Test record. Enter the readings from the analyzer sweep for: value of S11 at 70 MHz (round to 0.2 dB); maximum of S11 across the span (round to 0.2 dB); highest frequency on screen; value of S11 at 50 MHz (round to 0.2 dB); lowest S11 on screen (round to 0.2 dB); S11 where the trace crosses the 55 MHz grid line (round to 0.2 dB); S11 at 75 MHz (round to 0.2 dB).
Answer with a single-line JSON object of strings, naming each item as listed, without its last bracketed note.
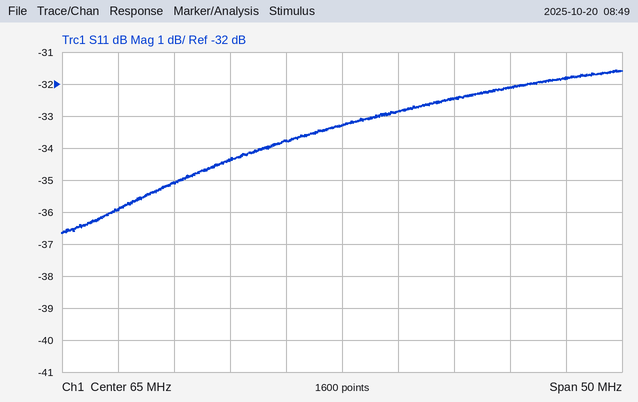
{"value of S11 at 70 MHz": "-32.8 dB", "maximum of S11 across the span": "-31.6 dB", "highest frequency on screen": "90 MHz", "value of S11 at 50 MHz": "-35.0 dB", "lowest S11 on screen": "-36.6 dB", "S11 where the trace crosses the 55 MHz grid line": "-34.4 dB", "S11 at 75 MHz": "-32.4 dB"}
